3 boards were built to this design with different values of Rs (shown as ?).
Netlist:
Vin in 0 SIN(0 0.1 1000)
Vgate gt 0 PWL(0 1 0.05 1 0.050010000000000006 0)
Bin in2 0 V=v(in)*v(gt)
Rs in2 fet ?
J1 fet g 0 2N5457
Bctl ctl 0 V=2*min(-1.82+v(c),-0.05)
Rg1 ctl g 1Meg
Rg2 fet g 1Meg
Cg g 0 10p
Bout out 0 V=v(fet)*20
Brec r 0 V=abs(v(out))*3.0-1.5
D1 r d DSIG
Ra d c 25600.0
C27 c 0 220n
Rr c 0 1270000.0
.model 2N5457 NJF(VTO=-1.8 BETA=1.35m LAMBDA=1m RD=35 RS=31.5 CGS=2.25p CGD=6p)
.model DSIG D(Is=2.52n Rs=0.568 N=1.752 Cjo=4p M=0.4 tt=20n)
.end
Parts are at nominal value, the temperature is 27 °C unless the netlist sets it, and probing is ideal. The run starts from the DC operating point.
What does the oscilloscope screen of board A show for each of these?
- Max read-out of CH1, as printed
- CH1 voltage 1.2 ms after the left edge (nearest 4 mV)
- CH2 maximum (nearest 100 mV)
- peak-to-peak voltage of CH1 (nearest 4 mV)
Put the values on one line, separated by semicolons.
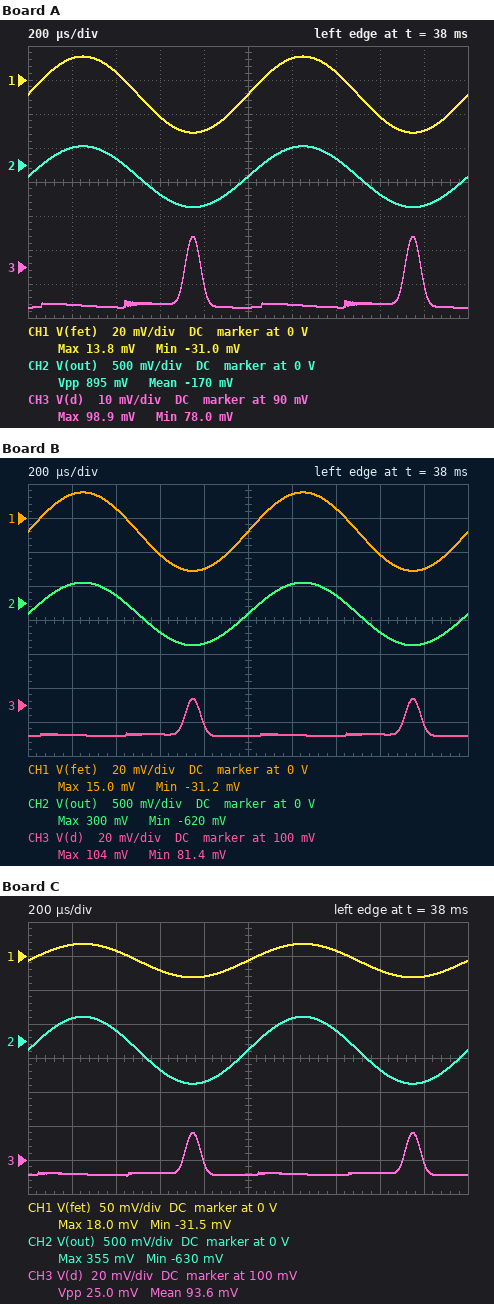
13.8 mV; 12 mV; 300 mV; 44 mV
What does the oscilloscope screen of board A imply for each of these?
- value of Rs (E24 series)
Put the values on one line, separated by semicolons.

22 kΩ
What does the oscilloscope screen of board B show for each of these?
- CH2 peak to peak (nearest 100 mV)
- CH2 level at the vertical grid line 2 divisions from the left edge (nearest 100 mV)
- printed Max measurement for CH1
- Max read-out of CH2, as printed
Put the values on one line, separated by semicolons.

900 mV; 100 mV; 15.0 mV; 300 mV
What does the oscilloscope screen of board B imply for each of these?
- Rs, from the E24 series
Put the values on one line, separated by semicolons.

20 kΩ
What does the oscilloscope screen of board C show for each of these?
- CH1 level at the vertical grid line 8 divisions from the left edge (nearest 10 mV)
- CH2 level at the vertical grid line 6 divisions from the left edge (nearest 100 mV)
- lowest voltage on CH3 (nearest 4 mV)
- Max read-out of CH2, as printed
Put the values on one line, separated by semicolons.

-20 mV; 300 mV; 92 mV; 355 mV
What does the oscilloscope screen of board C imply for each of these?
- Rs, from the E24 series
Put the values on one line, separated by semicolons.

16 kΩ
